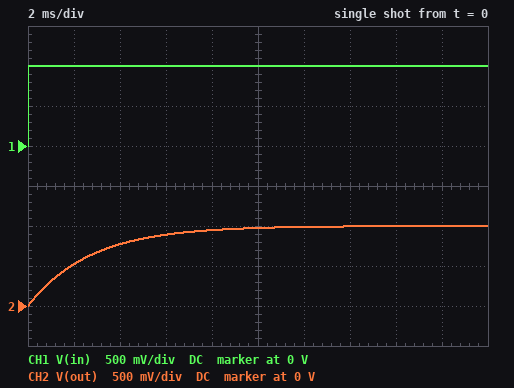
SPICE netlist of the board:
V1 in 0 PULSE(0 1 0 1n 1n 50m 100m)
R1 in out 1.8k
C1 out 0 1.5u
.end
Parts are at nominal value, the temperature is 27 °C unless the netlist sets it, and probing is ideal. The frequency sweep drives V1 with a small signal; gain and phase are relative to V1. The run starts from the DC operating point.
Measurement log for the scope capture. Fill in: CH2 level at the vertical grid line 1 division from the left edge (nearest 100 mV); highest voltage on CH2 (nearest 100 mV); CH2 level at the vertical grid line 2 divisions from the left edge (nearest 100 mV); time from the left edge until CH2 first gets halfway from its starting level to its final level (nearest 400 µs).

500 mV
1.0 V
800 mV
2.0 ms
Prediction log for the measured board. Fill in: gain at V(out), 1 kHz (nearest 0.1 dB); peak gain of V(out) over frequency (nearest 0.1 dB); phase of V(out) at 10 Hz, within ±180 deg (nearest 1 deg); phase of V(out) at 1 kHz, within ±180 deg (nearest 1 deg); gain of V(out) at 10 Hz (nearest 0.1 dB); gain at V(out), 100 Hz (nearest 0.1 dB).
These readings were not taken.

-24.6 dB
0 dB
-10 deg
-87 deg
-0.1 dB
-5.9 dB
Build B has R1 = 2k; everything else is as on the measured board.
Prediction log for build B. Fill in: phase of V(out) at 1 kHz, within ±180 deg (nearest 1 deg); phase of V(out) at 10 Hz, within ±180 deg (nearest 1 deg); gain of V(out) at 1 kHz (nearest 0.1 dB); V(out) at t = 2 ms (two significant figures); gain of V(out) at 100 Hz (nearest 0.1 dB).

-87 deg
-11 deg
-25.5 dB
490 mV
-6.6 dB
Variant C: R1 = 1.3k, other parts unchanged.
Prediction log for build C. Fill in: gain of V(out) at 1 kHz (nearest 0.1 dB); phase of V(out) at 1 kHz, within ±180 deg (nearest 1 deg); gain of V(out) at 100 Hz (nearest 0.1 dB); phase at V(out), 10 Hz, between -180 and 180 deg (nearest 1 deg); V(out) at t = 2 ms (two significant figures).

-21.8 dB
-85 deg
-4.0 dB
-7 deg
640 mV
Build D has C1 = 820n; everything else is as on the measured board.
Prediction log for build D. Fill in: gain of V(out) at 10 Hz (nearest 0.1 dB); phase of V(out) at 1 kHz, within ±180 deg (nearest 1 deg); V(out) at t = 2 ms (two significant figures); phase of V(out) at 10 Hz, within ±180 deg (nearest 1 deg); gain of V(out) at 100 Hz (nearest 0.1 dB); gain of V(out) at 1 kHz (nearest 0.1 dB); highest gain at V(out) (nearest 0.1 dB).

0 dB
-84 deg
740 mV
-5 deg
-2.7 dB
-19.4 dB
0 dB
